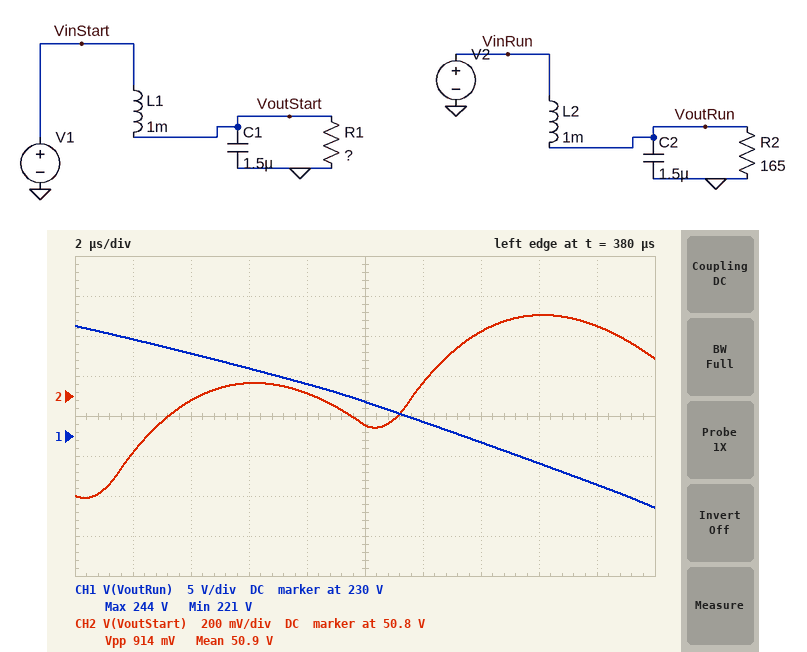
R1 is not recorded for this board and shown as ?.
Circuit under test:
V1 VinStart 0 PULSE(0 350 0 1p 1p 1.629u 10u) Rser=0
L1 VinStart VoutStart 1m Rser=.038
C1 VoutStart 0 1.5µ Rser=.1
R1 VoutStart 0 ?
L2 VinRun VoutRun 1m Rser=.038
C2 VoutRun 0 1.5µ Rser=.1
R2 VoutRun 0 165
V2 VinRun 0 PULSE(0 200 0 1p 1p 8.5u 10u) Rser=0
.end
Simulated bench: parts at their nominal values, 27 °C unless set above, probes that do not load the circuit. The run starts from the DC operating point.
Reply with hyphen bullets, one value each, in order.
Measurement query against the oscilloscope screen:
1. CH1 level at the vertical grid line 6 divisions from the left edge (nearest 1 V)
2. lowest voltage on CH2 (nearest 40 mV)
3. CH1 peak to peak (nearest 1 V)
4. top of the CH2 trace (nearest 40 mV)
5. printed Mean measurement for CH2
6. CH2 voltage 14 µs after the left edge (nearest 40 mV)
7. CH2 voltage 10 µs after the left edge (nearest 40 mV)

- 232 V
- 50.28 V
- 23 V
- 51.20 V
- 50.9 V
- 51.12 V
- 50.64 V
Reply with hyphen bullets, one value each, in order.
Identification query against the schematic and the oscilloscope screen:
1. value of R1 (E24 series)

- 5.6 Ω
